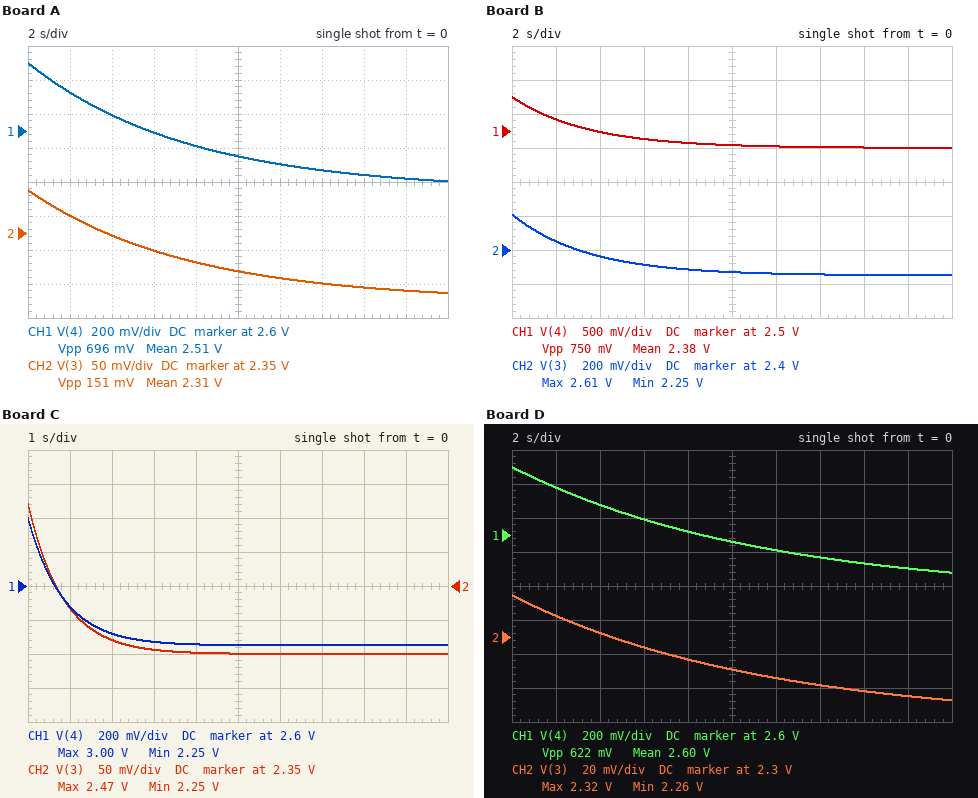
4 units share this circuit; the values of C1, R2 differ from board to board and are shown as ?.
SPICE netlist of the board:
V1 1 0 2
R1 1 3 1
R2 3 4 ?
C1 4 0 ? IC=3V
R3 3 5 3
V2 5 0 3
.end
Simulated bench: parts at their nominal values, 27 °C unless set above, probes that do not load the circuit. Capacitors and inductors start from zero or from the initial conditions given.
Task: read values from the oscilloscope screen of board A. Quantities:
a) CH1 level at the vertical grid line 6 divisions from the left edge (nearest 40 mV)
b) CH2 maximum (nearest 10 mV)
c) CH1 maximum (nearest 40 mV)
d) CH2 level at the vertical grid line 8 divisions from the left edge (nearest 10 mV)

2.40 V
2.41 V
3.00 V
2.27 V
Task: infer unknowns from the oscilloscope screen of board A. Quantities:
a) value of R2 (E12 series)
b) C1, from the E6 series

2.7 Ω
2.2 F
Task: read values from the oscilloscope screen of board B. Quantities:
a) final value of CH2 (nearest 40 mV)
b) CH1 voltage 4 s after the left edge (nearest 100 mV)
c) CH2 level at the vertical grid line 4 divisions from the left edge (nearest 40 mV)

2.24 V
2.5 V
2.28 V
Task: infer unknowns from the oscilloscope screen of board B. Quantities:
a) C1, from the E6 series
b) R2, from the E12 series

2.2 F
0.82 Ω
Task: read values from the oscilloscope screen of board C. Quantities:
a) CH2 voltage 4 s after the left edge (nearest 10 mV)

2.25 V
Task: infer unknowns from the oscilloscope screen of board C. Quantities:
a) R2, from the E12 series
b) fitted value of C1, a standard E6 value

1.8 Ω
330 mF
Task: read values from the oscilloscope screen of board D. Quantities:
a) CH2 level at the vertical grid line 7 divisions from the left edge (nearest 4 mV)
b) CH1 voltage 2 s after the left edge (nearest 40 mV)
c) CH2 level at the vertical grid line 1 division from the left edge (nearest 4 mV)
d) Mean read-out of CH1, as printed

2.272 V
2.88 V
2.312 V
2.60 V
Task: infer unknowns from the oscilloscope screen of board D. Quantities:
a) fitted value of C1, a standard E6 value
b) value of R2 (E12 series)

1.5 F
6.8 Ω
